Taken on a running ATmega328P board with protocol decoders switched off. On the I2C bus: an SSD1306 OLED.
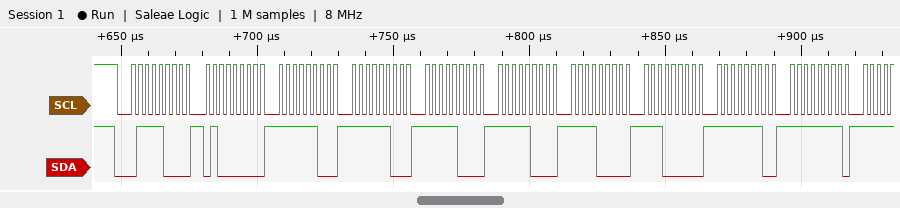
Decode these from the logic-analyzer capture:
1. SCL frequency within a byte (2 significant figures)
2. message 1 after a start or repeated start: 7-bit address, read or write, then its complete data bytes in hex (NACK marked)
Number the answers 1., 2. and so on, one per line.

1. 400 kHz
2. 0x3C write: 40 FC FC F8 F8 F0 E0 FE FF
